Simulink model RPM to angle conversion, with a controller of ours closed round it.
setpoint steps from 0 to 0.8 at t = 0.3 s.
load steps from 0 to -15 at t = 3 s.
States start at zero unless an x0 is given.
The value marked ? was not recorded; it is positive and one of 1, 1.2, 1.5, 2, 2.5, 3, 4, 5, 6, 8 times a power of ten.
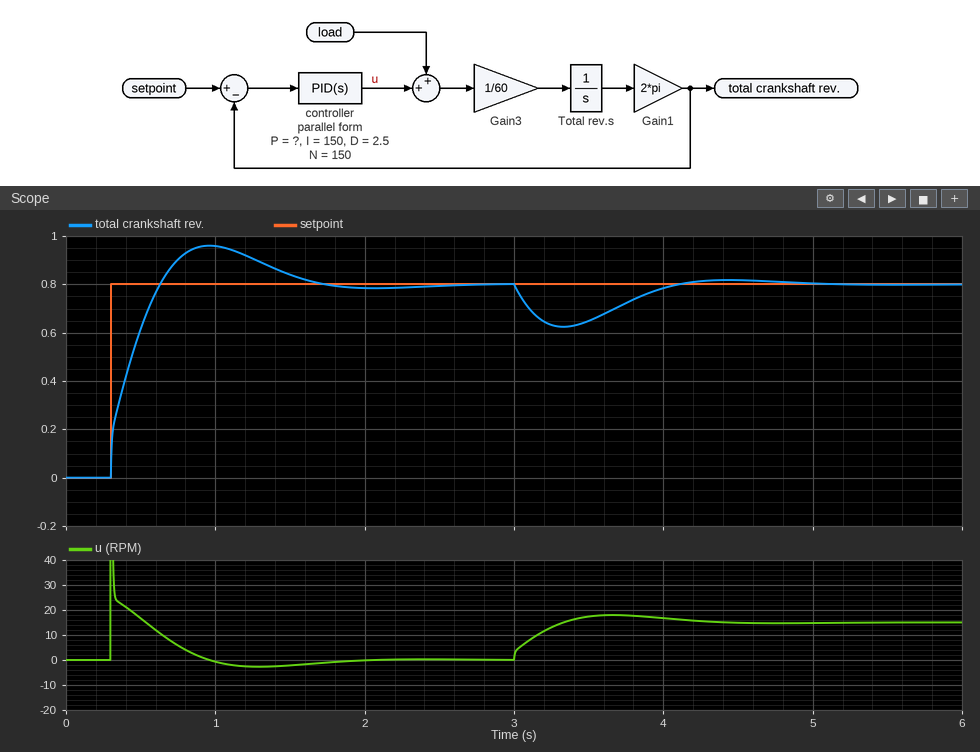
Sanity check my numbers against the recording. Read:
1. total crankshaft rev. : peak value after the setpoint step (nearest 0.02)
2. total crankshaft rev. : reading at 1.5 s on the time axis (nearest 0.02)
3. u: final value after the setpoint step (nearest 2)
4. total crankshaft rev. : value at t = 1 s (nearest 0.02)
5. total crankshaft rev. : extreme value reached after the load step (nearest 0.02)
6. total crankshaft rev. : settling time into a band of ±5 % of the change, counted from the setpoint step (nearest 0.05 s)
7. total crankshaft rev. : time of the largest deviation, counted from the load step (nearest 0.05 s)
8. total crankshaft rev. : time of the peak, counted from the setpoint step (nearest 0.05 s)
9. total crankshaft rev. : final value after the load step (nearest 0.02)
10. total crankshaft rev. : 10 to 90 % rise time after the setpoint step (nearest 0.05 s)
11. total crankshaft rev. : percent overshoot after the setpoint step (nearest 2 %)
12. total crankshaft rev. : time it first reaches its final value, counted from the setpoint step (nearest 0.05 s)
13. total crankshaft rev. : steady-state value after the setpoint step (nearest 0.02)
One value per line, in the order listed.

0.96
0.84
0
0.96
0.62
1.20 s
0.35 s
0.65 s
0.80
0.25 s
20 %
0.35 s
0.80
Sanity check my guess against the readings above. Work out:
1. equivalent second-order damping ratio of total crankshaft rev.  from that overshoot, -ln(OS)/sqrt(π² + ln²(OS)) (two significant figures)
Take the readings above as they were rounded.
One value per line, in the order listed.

0.46
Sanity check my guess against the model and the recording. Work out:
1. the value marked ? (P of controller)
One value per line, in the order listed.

50
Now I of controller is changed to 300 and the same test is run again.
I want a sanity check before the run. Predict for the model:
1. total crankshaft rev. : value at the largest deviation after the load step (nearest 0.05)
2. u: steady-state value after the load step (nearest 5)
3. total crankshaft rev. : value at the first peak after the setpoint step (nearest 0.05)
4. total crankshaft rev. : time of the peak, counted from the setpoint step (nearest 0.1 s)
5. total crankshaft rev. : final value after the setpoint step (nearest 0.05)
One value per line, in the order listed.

0.65
15
1.00
0.5 s
0.80
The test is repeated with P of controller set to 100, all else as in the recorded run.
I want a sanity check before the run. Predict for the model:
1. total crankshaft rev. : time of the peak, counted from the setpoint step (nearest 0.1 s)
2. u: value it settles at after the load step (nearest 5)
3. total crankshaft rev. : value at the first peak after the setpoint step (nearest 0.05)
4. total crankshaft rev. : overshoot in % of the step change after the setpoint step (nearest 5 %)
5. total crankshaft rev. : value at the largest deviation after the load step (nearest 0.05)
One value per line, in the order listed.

0.5 s
15
0.85
10 %
0.70
